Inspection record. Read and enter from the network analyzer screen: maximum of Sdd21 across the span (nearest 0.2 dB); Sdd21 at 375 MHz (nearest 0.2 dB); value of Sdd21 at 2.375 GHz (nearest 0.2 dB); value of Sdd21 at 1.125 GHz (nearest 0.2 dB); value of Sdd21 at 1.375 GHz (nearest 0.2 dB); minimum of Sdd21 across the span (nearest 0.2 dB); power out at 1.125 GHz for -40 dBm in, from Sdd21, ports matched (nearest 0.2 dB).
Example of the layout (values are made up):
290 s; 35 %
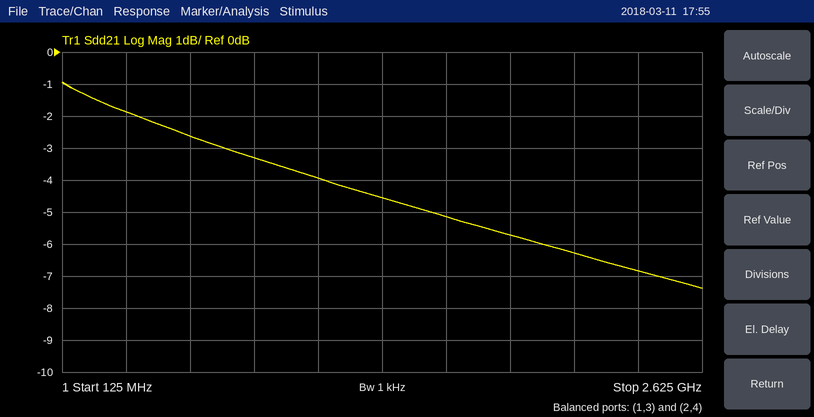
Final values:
-1.0 dB; -1.8 dB; -6.8 dB; -4.0 dB; -4.6 dB; -7.4 dB; -44.0 dBm
